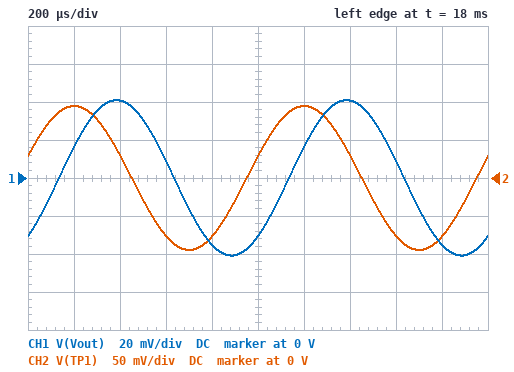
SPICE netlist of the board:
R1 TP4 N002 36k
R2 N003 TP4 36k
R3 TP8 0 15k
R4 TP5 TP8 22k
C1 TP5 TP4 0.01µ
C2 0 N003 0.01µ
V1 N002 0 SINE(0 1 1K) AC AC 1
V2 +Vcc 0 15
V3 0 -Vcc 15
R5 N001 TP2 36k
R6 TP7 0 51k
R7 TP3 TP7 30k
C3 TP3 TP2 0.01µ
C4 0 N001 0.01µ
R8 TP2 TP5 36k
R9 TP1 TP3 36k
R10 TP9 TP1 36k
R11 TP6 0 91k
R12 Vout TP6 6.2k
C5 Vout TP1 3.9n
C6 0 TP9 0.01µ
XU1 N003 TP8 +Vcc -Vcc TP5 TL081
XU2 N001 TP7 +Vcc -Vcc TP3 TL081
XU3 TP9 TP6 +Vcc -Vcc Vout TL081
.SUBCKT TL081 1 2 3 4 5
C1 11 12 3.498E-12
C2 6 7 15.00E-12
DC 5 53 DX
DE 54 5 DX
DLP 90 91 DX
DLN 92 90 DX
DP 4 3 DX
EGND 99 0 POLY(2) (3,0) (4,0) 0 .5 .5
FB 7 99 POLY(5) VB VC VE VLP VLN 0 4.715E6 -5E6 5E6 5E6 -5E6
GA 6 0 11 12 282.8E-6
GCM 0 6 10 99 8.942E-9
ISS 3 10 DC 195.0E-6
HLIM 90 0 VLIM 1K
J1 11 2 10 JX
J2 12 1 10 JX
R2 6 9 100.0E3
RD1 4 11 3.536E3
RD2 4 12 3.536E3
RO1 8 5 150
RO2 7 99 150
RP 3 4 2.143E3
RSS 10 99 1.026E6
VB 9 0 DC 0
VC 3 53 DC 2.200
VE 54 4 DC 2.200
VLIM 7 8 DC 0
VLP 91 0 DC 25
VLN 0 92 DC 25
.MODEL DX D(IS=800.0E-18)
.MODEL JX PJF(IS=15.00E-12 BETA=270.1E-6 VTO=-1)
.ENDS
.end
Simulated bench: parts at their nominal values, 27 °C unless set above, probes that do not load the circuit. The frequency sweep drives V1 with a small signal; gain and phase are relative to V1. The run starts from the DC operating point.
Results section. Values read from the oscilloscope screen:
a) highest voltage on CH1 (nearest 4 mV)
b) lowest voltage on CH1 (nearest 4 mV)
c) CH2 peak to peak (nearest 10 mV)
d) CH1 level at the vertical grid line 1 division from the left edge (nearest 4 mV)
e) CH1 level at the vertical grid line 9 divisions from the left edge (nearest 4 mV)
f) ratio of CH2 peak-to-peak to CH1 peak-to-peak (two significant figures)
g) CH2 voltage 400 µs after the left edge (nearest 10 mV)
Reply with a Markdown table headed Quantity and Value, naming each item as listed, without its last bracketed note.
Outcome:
| Quantity | Value |
|---|---|
| highest voltage on CH1 | 40 mV |
| lowest voltage on CH1 | -40 mV |
| CH2 peak to peak | 190 mV |
| CH1 level at the vertical grid line 1 division from the left edge | 16 mV |
| CH1 level at the vertical grid line 9 divisions from the left edge | -36 mV |
| ratio of CH2 peak-to-peak to CH1 peak-to-peak | 2.3 |
| CH2 voltage 400 µs after the left edge | 30 mV |
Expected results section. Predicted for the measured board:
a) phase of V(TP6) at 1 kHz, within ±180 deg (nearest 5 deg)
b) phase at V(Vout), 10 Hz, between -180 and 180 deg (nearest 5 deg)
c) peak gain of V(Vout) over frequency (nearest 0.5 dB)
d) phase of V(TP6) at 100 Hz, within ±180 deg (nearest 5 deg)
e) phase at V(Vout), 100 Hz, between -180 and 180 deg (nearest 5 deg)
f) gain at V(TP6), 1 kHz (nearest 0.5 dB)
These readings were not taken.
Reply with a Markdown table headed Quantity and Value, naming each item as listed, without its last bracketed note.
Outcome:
| Quantity | Value |
|---|---|
| phase of V(TP6) at 1 kHz, within ±180 deg | -50 deg |
| phase at V(Vout), 10 Hz, between -180 and 180 deg | -5 deg |
| peak gain of V(Vout) over frequency | 12.5 dB |
| phase of V(TP6) at 100 Hz, within ±180 deg | -50 deg |
| phase at V(Vout), 100 Hz, between -180 and 180 deg | -50 deg |
| gain at V(TP6), 1 kHz | -28.5 dB |
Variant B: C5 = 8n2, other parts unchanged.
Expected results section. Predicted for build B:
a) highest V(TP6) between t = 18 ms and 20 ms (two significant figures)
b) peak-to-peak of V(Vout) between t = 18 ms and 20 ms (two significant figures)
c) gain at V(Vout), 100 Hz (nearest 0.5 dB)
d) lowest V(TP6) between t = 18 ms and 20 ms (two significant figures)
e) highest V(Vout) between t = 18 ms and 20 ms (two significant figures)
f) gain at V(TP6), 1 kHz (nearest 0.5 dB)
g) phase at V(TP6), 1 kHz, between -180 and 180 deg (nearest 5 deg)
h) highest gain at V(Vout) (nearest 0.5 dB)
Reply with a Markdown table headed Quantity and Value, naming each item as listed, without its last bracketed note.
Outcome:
| Quantity | Value |
|---|---|
| highest V(TP6) between t = 18 ms and 20 ms | 32 mV |
| peak-to-peak of V(Vout) between t = 18 ms and 20 ms | 69 mV |
| gain at V(Vout), 100 Hz | 12.5 dB |
| lowest V(TP6) between t = 18 ms and 20 ms | -32 mV |
| highest V(Vout) between t = 18 ms and 20 ms | 34 mV |
| gain at V(TP6), 1 kHz | -30.0 dB |
| phase at V(TP6), 1 kHz, between -180 and 180 deg | -70 deg |
| highest gain at V(Vout) | 12.5 dB |
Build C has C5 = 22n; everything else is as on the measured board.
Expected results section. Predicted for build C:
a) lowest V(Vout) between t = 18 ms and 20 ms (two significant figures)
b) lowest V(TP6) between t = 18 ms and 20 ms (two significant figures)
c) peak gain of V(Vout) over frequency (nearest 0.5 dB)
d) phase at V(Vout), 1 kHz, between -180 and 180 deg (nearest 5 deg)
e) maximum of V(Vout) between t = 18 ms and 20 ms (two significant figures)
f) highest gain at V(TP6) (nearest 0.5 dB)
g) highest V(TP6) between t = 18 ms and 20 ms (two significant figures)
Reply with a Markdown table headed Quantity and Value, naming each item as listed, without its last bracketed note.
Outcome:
| Quantity | Value |
|---|---|
| lowest V(Vout) between t = 18 ms and 20 ms | -17 mV |
| lowest V(TP6) between t = 18 ms and 20 ms | -16 mV |
| peak gain of V(Vout) over frequency | 14.0 dB |
| phase at V(Vout), 1 kHz, between -180 and 180 deg | -105 deg |
| maximum of V(Vout) between t = 18 ms and 20 ms | 17 mV |
| highest gain at V(TP6) | 13.5 dB |
| highest V(TP6) between t = 18 ms and 20 ms | 16 mV |
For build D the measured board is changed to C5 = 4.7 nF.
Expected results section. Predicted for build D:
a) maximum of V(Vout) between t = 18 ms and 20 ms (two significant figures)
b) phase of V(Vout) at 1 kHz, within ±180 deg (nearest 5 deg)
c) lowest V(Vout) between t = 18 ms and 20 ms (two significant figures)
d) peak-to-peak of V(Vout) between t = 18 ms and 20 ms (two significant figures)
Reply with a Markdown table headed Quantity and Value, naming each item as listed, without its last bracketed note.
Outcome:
| Quantity | Value |
|---|---|
| maximum of V(Vout) between t = 18 ms and 20 ms | 40 mV |
| phase of V(Vout) at 1 kHz, within ±180 deg | -55 deg |
| lowest V(Vout) between t = 18 ms and 20 ms | -40 mV |
| peak-to-peak of V(Vout) between t = 18 ms and 20 ms | 80 mV |
